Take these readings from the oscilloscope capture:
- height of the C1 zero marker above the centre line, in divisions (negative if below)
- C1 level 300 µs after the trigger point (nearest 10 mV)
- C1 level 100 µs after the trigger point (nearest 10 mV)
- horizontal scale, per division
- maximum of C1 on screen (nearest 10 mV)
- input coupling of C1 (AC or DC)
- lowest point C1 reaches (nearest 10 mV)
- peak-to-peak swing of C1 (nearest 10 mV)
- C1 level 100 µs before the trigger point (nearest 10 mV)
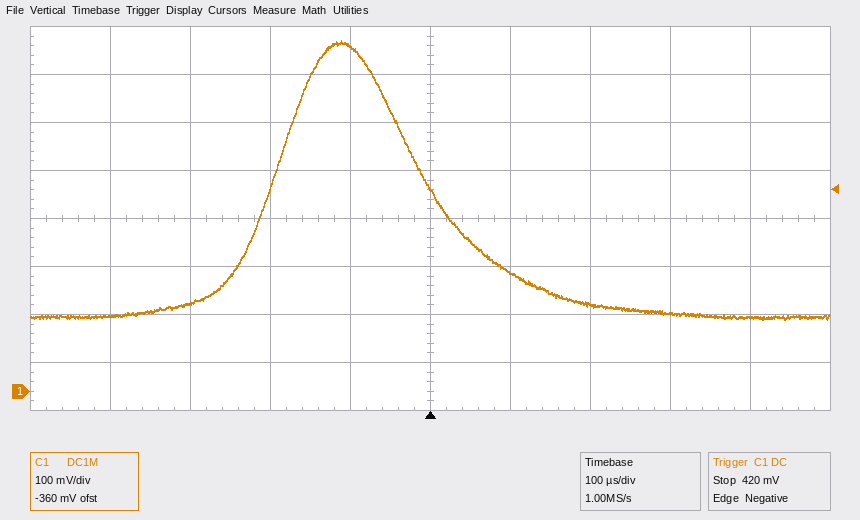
-3.6 div
160 mV
250 mV
100 µs
730 mV
DC
150 mV
580 mV
720 mV
